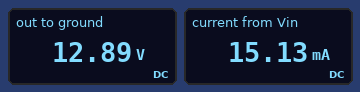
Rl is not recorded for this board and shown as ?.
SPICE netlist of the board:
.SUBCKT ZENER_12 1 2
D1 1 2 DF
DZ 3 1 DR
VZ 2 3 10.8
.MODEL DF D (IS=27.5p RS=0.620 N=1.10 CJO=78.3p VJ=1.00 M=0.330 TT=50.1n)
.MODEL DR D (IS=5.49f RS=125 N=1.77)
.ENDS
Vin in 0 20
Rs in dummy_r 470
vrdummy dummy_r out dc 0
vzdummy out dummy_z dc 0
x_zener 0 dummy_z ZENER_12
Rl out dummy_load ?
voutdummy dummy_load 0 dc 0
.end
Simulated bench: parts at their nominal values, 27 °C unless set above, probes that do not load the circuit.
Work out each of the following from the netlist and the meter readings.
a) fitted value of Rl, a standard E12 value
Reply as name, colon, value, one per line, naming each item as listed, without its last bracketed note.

fitted value of Rl, a standard E12 value: 1.5 kΩ
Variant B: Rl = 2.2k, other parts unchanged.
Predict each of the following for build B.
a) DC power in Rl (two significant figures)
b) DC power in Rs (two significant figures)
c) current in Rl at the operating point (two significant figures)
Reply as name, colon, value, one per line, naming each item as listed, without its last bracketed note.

DC power in Rl: 79 mW
DC power in Rs: 100 mW
current in Rl at the operating point: 6.0 mA
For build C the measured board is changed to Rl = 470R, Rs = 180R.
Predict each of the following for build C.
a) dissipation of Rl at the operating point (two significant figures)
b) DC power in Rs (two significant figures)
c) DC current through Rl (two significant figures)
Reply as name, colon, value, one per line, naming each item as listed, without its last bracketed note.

dissipation of Rl at the operating point: 370 mW
DC power in Rs: 250 mW
DC current through Rl: 28 mA
